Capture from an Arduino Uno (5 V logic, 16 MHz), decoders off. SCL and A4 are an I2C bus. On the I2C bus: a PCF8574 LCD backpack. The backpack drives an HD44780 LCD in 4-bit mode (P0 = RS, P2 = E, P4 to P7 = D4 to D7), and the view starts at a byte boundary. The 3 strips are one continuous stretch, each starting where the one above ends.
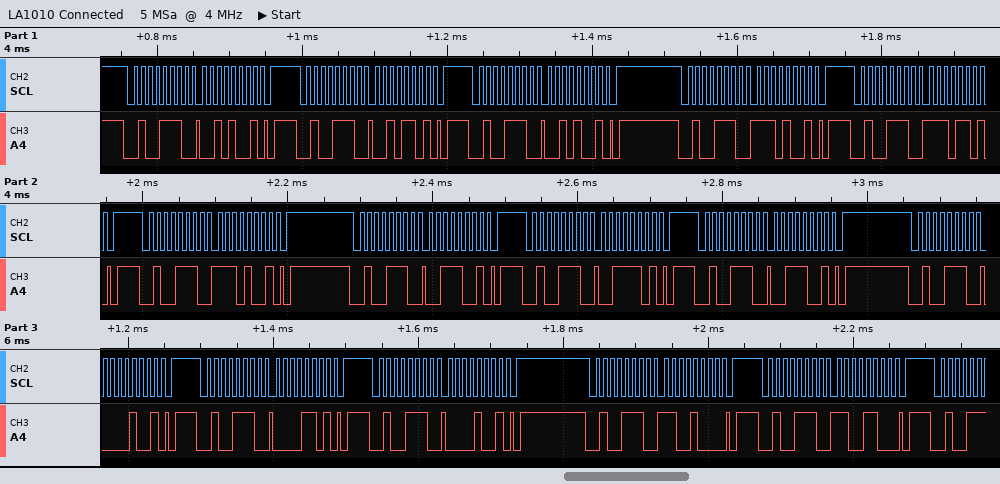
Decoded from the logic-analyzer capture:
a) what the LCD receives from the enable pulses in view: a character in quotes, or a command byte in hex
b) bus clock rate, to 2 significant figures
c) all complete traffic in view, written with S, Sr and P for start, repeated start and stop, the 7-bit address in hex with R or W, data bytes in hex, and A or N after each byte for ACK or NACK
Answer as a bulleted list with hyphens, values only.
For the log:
- '.' '0'
- 100 kHz
- S 27W A 29 A P S 27W A 2D A P S 27W A 29 A P S 27W A E9 A P S 27W A ED A P S 27W A E9 A P S 27W A 39 A P S 27W A 3D A P S 27W A 39 A P S 27W A 09 A P S 27W A 0D A P S 27W A 09 A P S 27W A C8 A P S 27W A CC A P
